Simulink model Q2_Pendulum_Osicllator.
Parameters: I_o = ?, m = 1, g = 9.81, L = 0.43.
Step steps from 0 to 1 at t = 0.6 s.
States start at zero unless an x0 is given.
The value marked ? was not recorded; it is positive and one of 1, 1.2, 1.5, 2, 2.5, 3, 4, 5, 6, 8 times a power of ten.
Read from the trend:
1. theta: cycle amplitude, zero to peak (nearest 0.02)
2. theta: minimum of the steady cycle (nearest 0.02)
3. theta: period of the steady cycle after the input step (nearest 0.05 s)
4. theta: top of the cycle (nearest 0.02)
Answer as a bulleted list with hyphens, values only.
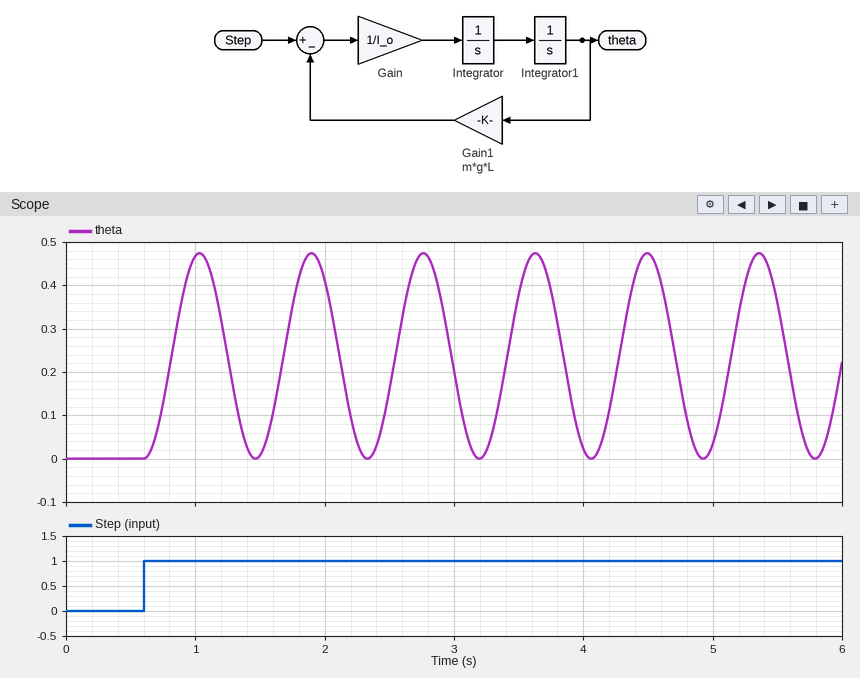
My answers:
- 0.24
- 0.00
- 0.85 s
- 0.48
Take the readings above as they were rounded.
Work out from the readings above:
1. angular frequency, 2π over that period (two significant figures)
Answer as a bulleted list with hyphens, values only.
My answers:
- 7.4 rad/s
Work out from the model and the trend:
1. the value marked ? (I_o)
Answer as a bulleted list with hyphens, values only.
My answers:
- 0.08
